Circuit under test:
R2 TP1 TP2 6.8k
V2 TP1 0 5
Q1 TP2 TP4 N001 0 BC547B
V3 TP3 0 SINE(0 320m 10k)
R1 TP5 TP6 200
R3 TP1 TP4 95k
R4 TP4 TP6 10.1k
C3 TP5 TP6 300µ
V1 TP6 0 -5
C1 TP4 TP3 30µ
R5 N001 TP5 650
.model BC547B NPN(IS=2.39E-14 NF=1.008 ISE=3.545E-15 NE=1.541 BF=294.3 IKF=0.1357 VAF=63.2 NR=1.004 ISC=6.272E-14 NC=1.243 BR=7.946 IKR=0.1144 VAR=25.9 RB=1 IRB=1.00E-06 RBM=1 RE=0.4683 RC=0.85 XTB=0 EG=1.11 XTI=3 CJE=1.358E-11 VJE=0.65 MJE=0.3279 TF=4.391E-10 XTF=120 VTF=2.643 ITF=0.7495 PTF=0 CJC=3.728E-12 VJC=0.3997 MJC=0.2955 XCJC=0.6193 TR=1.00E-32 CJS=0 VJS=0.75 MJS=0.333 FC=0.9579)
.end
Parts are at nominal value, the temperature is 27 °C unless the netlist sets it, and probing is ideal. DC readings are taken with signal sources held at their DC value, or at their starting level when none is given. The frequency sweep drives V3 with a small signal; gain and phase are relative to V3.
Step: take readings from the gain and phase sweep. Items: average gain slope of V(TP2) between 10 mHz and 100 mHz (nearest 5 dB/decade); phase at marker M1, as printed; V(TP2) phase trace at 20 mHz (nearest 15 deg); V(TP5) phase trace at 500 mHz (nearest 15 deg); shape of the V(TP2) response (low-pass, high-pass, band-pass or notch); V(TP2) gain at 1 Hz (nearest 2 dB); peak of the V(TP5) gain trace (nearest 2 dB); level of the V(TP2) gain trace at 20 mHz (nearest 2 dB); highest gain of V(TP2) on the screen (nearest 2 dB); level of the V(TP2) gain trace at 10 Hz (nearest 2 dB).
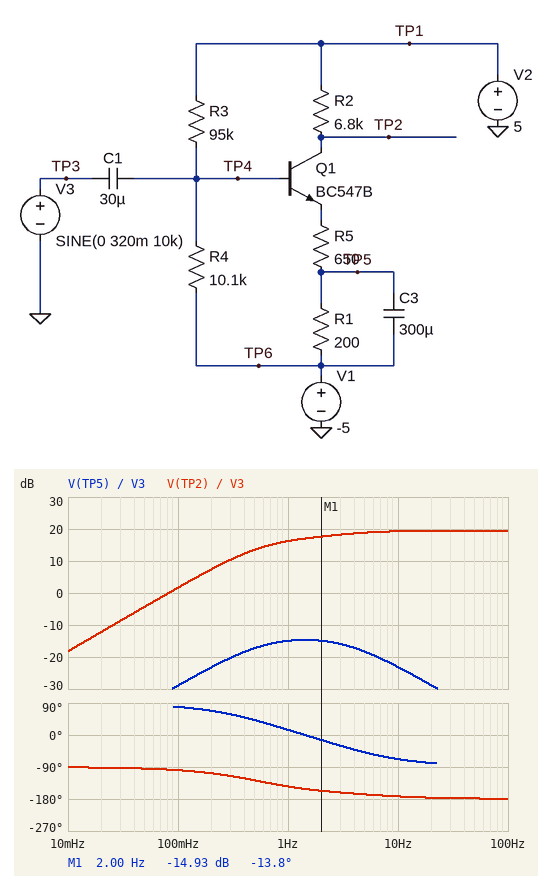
20 dB/decade
-13.8 deg
-90 deg
45 deg
high-pass
16 dB
-14 dB
-12 dB
20 dB
20 dB
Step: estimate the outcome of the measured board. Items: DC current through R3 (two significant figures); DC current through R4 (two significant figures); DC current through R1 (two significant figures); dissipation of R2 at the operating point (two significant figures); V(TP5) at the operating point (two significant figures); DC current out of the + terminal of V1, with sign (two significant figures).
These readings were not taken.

95 µA
94 µA
400 µA
1.1 mW
-4.9 V
-490 µA
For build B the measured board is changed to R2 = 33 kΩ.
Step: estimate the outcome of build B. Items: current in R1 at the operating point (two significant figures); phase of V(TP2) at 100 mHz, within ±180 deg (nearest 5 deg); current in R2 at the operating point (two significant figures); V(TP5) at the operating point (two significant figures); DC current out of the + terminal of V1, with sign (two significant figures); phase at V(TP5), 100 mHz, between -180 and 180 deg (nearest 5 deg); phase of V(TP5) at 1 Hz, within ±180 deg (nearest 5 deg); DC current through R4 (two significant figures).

300 µA
-90 deg
290 µA
-4.9 V
-390 µA
85 deg
55 deg
86 µA
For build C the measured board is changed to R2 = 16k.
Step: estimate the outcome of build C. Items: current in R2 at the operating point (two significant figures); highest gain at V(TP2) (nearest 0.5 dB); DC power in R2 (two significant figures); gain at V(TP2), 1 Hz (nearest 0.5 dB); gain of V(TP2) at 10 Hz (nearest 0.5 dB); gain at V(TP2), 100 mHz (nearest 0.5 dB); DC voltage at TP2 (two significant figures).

390 µA
27.0 dB
2.5 mW
23.5 dB
26.5 dB
9.0 dB
-1.3 V
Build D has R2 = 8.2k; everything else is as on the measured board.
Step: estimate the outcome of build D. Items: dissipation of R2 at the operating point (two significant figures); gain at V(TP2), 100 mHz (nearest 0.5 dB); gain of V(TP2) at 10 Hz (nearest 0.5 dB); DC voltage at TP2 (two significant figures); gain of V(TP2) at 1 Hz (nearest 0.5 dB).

1.3 mW
3.5 dB
21.0 dB
1.8 V
18.0 dB
